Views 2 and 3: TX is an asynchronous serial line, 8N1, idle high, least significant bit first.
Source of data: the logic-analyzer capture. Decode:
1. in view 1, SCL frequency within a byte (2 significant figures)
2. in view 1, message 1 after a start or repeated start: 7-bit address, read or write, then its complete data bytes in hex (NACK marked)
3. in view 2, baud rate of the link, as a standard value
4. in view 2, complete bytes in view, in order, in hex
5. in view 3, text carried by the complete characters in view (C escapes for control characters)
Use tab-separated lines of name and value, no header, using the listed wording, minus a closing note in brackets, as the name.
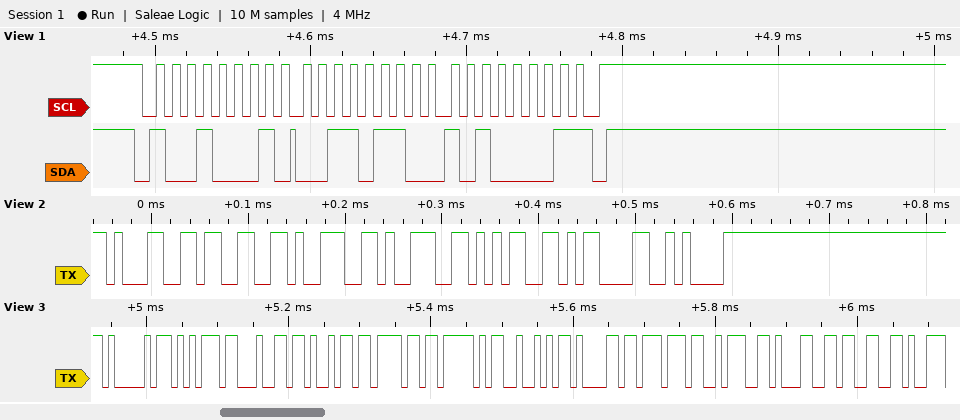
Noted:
in view 1, SCL frequency within a byte	100 kHz
in view 1, message 1 after a start or repeated start: 7-bit address, read or write, then its complete data bytes in hex	0x48 read: 36 A1 NACK
in view 2, baud rate of the link, as a standard value	115200 baud
in view 2, complete bytes in view, in order, in hex	31 33 39 39 35 0D 0A
in view 3, text carried by the complete characters in view	"Audio_Raw:13"
